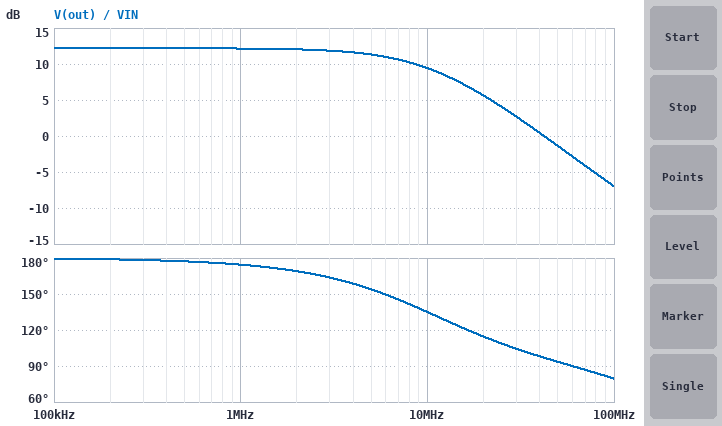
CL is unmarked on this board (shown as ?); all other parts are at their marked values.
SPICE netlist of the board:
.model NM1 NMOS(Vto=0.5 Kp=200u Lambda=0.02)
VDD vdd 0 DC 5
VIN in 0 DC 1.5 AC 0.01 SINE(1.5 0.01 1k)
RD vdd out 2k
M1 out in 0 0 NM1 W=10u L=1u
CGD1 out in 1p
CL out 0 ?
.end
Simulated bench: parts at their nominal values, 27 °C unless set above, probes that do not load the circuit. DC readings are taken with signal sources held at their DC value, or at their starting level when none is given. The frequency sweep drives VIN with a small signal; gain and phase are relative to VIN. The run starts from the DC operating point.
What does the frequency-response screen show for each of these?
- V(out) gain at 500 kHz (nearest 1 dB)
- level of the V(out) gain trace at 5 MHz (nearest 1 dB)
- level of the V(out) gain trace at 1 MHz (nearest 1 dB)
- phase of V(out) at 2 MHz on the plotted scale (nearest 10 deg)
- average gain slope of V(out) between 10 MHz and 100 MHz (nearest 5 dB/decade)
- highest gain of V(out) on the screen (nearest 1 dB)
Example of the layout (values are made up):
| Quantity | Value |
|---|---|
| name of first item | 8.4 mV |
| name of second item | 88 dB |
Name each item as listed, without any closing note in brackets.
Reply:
| Quantity | Value |
|---|---|
| V(out) gain at 500 kHz | 12 dB |
| level of the V(out) gain trace at 5 MHz | 11 dB |
| level of the V(out) gain trace at 1 MHz | 12 dB |
| phase of V(out) at 2 MHz on the plotted scale | 170 deg |
| average gain slope of V(out) between 10 MHz and 100 MHz | -15 dB/decade |
| highest gain of V(out) on the screen | 12 dB |
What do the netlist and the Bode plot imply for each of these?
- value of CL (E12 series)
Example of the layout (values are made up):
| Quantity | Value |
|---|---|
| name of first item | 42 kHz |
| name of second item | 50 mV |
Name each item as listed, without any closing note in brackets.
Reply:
| Quantity | Value |
|---|---|
| value of CL | 6.8 pF |
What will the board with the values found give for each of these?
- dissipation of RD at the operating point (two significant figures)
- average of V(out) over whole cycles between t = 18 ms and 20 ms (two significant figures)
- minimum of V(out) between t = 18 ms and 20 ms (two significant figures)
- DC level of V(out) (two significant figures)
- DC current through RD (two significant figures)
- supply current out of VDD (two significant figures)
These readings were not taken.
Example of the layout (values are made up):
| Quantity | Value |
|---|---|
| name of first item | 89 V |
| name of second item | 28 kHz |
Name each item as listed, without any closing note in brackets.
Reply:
| Quantity | Value |
|---|---|
| dissipation of RD at the operating point | 2.2 mW |
| average of V(out) over whole cycles between t = 18 ms and 20 ms | 2.9 V |
| minimum of V(out) between t = 18 ms and 20 ms | 2.8 V |
| DC level of V(out) | 2.9 V |
| DC current through RD | 1.1 mA |
| supply current out of VDD | 1.1 mA |
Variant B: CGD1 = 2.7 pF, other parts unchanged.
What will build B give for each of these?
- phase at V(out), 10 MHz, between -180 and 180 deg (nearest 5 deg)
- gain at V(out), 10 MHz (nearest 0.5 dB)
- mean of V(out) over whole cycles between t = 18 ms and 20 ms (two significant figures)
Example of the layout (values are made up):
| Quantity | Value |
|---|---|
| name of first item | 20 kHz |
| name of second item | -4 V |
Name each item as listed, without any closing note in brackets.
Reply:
| Quantity | Value |
|---|---|
| phase at V(out), 10 MHz, between -180 and 180 deg | 125 deg |
| gain at V(out), 10 MHz | 8.5 dB |
| mean of V(out) over whole cycles between t = 18 ms and 20 ms | 2.9 V |
